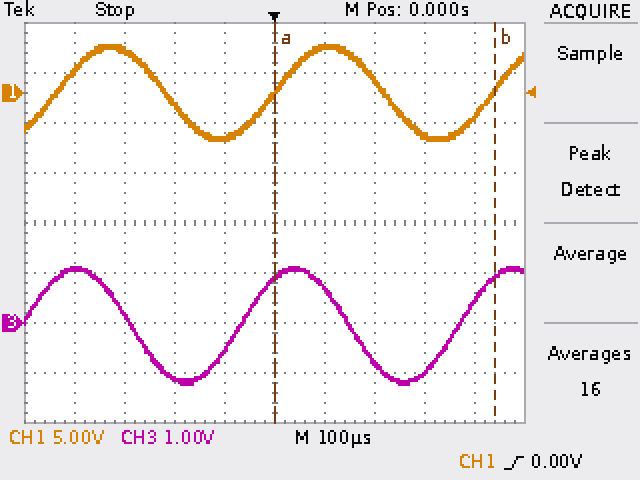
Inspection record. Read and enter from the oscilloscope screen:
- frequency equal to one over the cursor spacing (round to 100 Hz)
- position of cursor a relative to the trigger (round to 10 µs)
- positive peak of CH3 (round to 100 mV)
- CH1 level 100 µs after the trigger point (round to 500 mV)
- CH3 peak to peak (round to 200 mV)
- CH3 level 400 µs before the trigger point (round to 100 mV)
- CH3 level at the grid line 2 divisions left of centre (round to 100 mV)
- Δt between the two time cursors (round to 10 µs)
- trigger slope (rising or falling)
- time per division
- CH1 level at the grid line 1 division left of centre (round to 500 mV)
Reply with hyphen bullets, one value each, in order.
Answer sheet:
- 2.3 kHz
- 0 µs
- 1.1 V
- 4.5 V
- 2.4 V
- 1.1 V
- -1.1 V
- 440 µs
- rising
- 100 µs
- -4.5 V
